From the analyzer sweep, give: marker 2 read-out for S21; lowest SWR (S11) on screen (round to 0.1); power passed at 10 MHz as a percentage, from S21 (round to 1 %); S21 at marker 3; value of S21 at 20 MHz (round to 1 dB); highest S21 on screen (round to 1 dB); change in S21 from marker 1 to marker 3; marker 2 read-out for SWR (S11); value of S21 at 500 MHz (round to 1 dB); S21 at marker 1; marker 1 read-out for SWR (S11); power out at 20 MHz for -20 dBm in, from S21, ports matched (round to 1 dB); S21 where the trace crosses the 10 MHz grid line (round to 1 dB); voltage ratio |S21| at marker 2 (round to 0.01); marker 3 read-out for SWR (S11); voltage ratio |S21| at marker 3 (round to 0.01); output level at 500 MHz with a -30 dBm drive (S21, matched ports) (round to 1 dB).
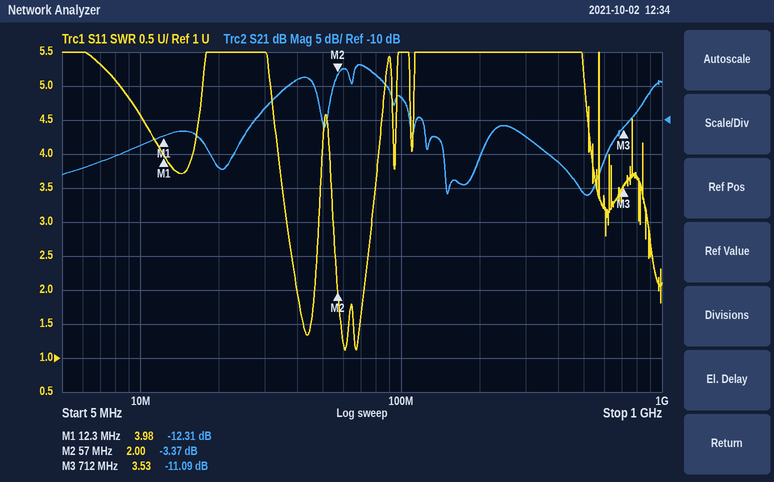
-3.37 dB
1.1
4 %
-11.09 dB
-17 dB
-2 dB
1.22 dB
2.00
-21 dB
-12.31 dB
3.98
-37 dBm
-14 dB
0.68
3.53
0.28
-51 dBm
